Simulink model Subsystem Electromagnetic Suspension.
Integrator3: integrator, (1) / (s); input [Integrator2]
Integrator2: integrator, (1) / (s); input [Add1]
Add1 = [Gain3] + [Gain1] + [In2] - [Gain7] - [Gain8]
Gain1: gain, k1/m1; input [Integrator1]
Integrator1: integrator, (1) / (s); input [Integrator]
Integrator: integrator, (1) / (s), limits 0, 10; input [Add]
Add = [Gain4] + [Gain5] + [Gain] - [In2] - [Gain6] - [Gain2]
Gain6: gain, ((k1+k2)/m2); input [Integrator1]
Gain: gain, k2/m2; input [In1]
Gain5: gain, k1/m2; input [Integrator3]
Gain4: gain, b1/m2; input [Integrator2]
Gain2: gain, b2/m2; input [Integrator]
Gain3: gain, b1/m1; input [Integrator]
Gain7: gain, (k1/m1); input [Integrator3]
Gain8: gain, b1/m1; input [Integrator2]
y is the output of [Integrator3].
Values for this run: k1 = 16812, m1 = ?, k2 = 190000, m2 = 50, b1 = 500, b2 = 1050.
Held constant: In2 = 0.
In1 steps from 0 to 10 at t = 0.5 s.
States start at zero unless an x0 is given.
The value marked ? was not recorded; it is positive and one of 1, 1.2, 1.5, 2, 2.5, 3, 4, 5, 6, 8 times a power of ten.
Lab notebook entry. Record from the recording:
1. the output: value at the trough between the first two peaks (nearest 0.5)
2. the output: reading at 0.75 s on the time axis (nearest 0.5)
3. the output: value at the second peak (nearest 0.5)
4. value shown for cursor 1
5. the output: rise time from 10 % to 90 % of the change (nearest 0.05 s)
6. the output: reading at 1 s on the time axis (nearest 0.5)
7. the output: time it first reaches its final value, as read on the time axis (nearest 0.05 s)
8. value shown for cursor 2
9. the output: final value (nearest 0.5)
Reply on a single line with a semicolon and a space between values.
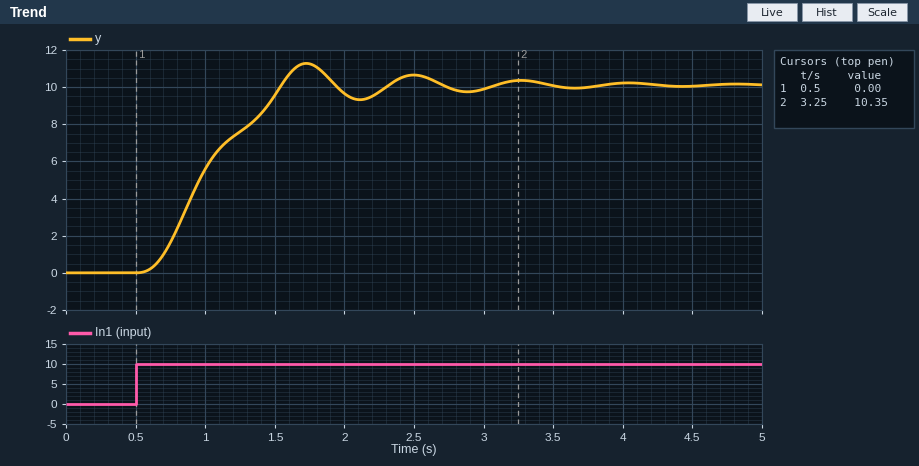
9.5; 1.5; 10.5; 0.00; 0.75 s; 5.5; 1.55 s; 10.35; 10.0
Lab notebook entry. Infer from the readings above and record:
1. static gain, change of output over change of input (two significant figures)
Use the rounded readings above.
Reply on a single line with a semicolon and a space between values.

1.0
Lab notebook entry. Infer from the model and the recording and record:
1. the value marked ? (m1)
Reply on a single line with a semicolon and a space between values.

250
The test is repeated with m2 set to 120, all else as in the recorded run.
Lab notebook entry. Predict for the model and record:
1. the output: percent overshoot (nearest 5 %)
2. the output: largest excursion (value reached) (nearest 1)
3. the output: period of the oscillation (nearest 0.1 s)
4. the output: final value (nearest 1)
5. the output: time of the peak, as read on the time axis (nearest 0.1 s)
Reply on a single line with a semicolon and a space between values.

10 %; 11; 0.8 s; 10; 1.7 s
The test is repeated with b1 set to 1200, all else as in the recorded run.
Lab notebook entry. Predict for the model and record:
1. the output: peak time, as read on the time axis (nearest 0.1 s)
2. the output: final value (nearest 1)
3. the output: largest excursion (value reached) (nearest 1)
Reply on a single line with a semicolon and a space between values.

1.7 s; 10; 11
